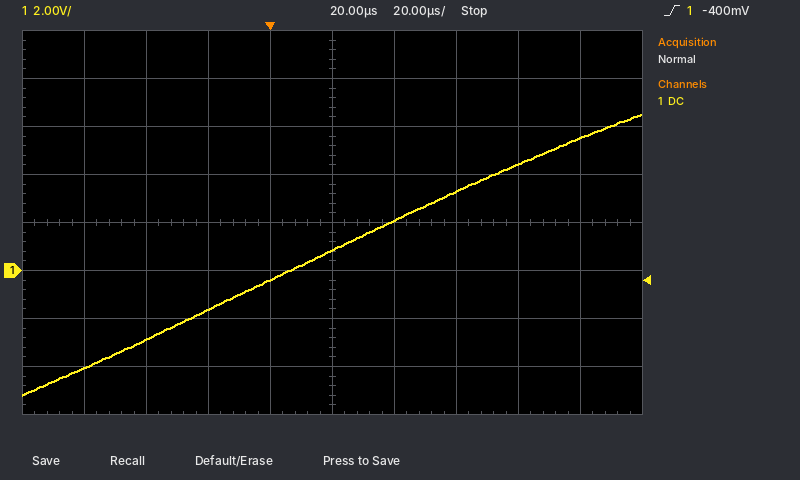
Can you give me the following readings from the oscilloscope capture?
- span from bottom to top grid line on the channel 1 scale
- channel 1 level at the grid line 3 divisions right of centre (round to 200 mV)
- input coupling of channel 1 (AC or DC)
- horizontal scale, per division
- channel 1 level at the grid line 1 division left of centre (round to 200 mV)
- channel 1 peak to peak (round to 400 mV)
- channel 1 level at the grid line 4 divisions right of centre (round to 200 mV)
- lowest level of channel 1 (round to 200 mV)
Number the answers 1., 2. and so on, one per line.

1. 16 V
2. 4.4 V
3. DC
4. 20 µs
5. -400 mV
6. 11.6 V
7. 5.6 V
8. -5.2 V
